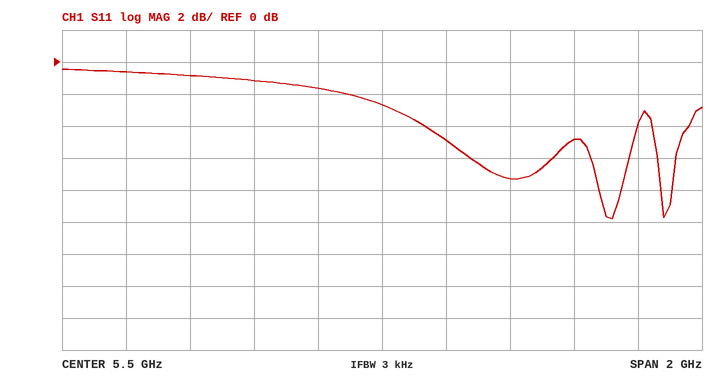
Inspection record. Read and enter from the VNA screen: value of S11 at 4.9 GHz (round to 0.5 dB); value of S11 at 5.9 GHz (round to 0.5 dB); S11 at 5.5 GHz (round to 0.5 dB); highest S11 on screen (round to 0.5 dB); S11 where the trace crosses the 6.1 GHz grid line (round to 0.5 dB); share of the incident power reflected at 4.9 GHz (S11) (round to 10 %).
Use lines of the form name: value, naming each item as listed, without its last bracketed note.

value of S11 at 4.9 GHz: -1.0 dB
value of S11 at 5.9 GHz: -7.5 dB
S11 at 5.5 GHz: -2.5 dB
highest S11 on screen: -0.5 dB
S11 where the trace crosses the 6.1 GHz grid line: -5.0 dB
share of the incident power reflected at 4.9 GHz (S11): 80 %
